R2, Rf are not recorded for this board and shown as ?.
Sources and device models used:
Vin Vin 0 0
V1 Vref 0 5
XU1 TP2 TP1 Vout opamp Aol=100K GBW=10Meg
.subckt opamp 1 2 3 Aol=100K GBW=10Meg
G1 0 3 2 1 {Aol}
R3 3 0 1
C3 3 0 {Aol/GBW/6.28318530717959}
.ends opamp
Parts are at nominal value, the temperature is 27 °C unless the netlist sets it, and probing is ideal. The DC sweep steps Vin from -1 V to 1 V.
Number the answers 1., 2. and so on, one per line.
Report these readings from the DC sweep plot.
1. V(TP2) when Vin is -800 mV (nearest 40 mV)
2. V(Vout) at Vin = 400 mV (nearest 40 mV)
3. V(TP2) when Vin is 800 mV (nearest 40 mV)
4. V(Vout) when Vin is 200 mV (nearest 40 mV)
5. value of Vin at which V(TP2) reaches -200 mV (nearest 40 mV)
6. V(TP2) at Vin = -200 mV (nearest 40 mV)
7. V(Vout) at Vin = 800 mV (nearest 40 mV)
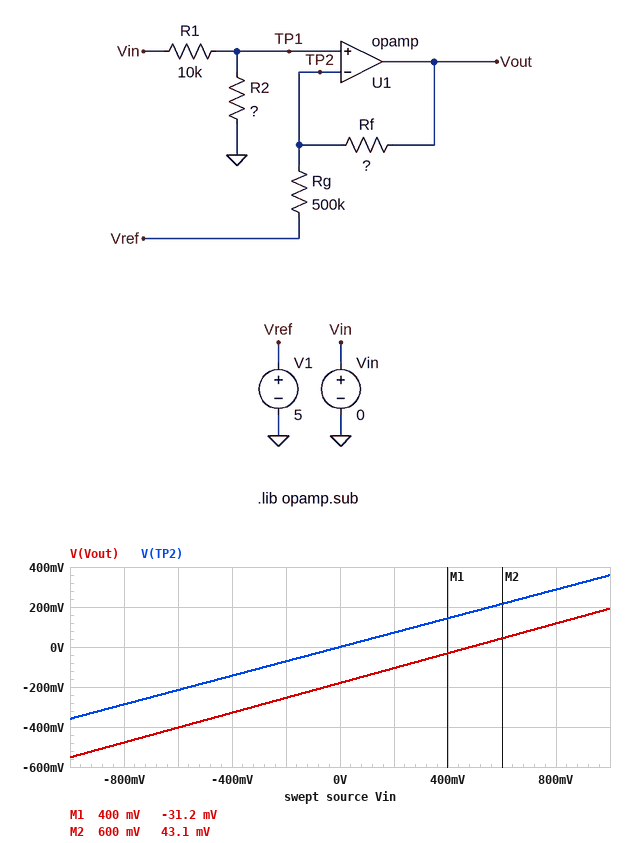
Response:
1. -280 mV
2. -40 mV
3. 280 mV
4. -120 mV
5. -560 mV
6. -80 mV
7. 120 mV
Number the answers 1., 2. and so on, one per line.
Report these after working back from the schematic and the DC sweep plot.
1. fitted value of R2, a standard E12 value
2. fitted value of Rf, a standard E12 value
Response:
1. 5.6 kΩ
2. 18 kΩ
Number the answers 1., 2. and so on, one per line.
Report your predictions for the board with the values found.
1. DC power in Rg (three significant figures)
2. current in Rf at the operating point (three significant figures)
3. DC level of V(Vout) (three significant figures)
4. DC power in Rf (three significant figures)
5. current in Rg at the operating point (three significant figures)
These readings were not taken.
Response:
1. 50.0 µW
2. 10.0 µA
3. -180 mV
4. 1.80 µW
5. 10.0 µA
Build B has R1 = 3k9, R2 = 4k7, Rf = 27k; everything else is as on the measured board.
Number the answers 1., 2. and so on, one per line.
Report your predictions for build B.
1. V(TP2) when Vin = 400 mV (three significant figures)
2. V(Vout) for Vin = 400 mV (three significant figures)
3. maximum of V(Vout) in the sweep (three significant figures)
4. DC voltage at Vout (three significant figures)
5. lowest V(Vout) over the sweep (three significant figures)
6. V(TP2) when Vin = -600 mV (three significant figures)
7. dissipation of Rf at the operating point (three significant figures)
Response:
1. 219 mV
2. -39.6 mV
3. 306 mV
4. -270 mV
5. -846 mV
6. -328 mV
7. 2.70 µW
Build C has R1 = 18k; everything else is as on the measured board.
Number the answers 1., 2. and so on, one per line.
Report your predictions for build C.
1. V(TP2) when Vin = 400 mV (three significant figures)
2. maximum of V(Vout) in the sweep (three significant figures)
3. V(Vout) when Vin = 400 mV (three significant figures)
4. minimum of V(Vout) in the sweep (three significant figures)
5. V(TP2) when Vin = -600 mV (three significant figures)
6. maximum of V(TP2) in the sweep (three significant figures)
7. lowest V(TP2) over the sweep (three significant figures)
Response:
1. 94.9 mV
2. 65.8 mV
3. -81.7 mV
4. -426 mV
5. -142 mV
6. 237 mV
7. -237 mV
